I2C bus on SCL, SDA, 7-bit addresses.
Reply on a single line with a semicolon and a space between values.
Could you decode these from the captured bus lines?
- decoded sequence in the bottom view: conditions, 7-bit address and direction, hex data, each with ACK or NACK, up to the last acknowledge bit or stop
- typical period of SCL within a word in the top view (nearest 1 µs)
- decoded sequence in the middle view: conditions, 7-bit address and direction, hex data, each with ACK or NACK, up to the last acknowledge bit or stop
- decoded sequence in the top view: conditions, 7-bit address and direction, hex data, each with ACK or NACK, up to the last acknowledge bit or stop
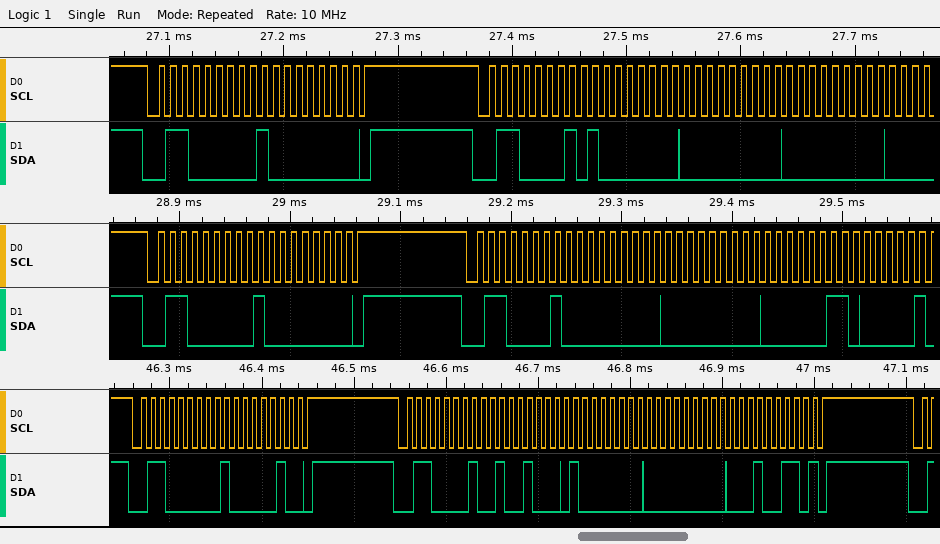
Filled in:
start, address 30 write ACK, 82 ACK, stop, start, address 30 read ACK, 48 ACK, 80 ACK, 00 ACK, 26 NACK, stop; 10 µs; start, address 30 write ACK, 80 ACK, stop, start, address 30 read ACK, 00 ACK, 00 ACK, 06 ACK; start, address 30 write ACK, 80 ACK, stop, start, address 30 read ACK, 80 ACK, 00 ACK, 00 ACK
